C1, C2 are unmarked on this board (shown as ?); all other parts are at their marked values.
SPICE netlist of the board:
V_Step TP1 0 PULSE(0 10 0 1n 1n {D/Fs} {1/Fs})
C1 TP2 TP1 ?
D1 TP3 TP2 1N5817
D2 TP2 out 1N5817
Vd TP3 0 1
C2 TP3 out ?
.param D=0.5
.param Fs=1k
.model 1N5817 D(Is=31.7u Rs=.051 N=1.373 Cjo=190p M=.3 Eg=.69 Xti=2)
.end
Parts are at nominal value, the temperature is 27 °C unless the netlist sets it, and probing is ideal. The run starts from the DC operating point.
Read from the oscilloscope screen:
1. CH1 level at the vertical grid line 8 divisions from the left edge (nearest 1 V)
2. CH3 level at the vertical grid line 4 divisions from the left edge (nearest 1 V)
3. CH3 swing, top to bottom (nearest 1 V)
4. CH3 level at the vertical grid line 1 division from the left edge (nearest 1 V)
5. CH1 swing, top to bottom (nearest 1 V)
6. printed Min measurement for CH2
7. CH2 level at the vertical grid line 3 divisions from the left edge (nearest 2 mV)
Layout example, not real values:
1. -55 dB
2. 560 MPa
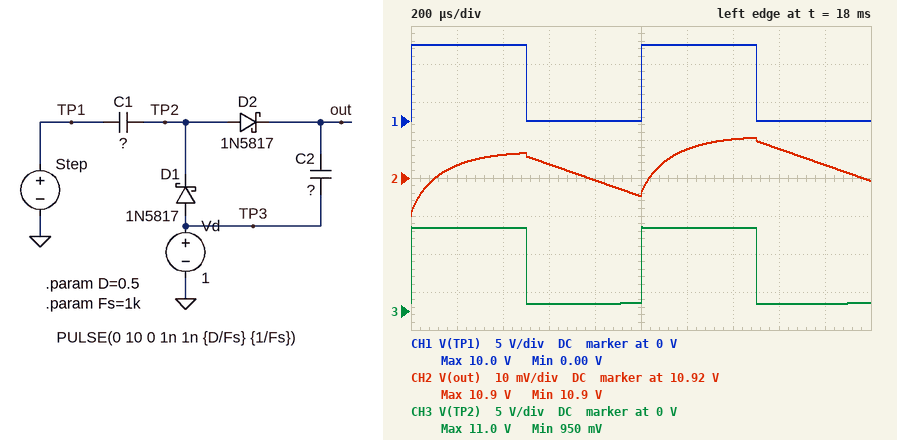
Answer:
1. 0 V
2. 1 V
3. 10 V
4. 11 V
5. 10 V
6. 10.9 V
7. 10.924 V
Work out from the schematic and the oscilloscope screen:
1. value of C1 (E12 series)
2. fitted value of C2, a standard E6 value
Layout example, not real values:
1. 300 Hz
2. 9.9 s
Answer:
1. 680 nF
2. 1.5 µF
